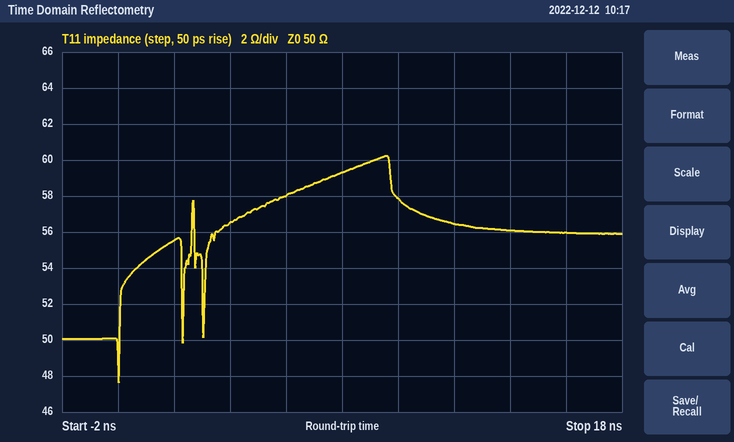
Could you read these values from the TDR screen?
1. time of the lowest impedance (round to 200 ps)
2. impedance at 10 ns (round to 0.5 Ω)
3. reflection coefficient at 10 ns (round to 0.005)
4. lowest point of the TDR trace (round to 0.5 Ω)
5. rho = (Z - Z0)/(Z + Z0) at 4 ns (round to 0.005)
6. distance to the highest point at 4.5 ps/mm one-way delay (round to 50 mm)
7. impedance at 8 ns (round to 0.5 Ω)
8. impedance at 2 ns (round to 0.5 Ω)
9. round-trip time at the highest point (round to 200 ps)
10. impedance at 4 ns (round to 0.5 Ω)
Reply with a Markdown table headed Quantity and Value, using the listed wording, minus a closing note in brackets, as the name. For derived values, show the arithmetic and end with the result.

| Quantity | Value |
|---|---|
| time of the lowest impedance | 0.0 ns |
| impedance at 10 ns | 58.0 Ω |
| reflection coefficient at 10 ns | (58 − 50)/(58 + 50) ≈ +0.0741, so +0.075 to the nearest 0.005 |
| lowest point of the TDR trace | 47.5 Ω |
| rho = (Z - Z0)/(Z + Z0) at 4 ns | (56.5 − 50)/(56.5 + 50) ≈ +0.0610, so +0.060 to the nearest 0.005 |
| distance to the highest point at 4.5 ps/mm one-way delay | 9.6 ns / 2 / 4.5 ps/mm ≈ 1.07 m, so 1.05 m to the nearest 50 mm |
| impedance at 8 ns | 59.5 Ω |
| impedance at 2 ns | 55.5 Ω |
| round-trip time at the highest point | 9.6 ns |
| impedance at 4 ns | 56.5 Ω |
